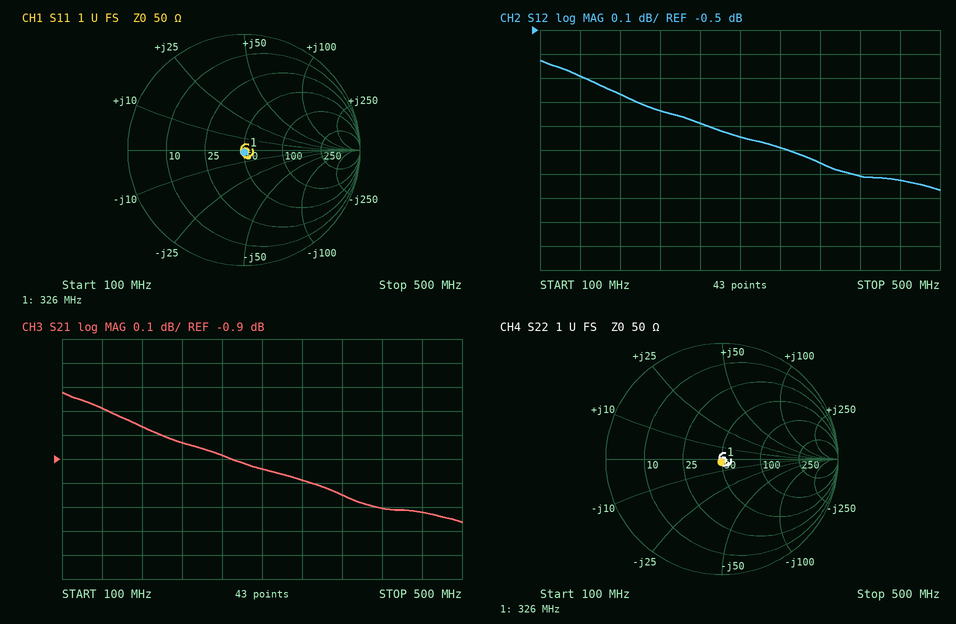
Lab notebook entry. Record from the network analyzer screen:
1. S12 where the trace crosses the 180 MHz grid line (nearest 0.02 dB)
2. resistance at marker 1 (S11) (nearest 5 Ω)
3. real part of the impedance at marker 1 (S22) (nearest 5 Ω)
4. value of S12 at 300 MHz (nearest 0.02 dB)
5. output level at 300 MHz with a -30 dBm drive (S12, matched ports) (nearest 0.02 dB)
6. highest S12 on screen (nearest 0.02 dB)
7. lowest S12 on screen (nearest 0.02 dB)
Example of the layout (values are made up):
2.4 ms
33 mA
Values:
-0.76 dB
50 Ω
50 Ω
-0.94 dB
-30.94 dBm
-0.62 dB
-1.16 dB
